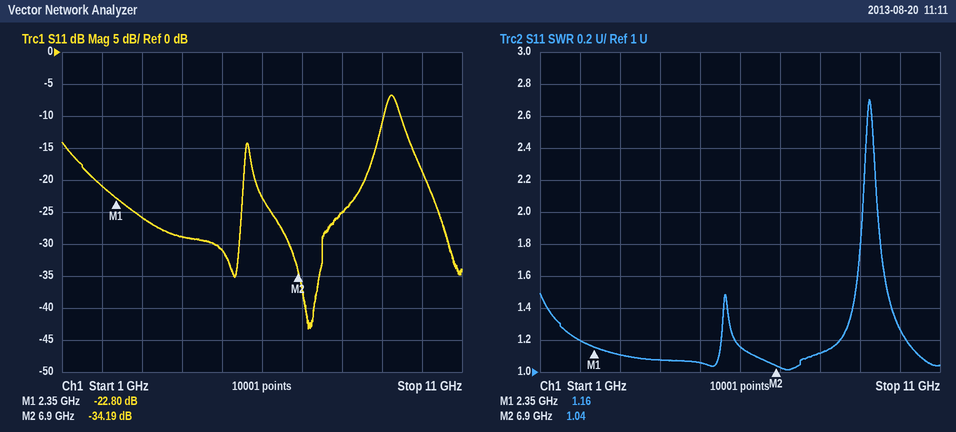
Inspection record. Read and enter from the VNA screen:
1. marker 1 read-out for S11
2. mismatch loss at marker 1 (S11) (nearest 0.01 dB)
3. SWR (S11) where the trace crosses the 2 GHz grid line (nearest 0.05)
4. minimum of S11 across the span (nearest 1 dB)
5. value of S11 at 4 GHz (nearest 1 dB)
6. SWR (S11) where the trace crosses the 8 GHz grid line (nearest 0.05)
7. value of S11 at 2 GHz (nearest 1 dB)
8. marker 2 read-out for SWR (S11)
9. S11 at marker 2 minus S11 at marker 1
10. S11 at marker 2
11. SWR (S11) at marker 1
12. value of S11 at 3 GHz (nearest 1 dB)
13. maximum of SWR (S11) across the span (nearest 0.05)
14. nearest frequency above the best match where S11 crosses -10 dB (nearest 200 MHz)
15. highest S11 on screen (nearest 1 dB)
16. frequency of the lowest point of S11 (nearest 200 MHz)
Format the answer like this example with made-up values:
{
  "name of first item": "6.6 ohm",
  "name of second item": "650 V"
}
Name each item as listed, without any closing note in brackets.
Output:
{
  "marker 1 read-out for S11": "-22.80 dB",
  "mismatch loss at marker 1 (S11)": "0.02 dB",
  "SWR (S11) where the trace crosses the 2 GHz grid line": "1.20",
  "minimum of S11 across the span": "-43 dB",
  "value of S11 at 4 GHz": "-29 dB",
  "SWR (S11) where the trace crosses the 8 GHz grid line": "1.10",
  "value of S11 at 2 GHz": "-21 dB",
  "marker 2 read-out for SWR": "1.04",
  "S11 at marker 2 minus S11 at marker 1": "-11.39 dB",
  "S11 at marker 2": "-34.19 dB",
  "SWR (S11) at marker 1": "1.16",
  "value of S11 at 3 GHz": "-26 dB",
  "maximum of SWR (S11) across the span": "2.70",
  "nearest frequency above the best match where S11 crosses -10 dB": "9.0 GHz",
  "highest S11 on screen": "-7 dB",
  "frequency of the lowest point of S11": "7.2 GHz"
}
